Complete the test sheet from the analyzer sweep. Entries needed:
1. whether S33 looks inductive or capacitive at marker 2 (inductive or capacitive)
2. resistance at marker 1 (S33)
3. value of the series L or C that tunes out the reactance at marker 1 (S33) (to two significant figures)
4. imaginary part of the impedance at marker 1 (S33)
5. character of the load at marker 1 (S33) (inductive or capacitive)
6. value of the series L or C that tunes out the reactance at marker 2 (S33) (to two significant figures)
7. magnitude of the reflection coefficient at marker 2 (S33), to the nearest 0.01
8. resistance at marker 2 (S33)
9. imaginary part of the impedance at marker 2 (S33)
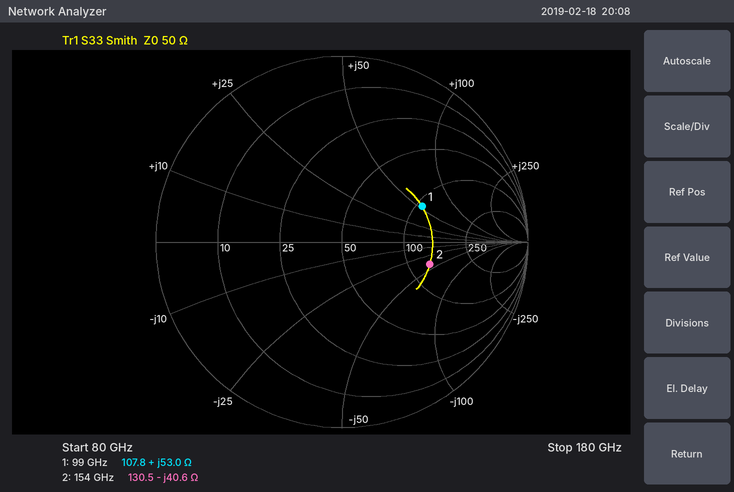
capacitive
107.8 Ω
30 fF
+53.0 Ω
inductive
42 pH
0.49
130.5 Ω
-40.6 Ω
